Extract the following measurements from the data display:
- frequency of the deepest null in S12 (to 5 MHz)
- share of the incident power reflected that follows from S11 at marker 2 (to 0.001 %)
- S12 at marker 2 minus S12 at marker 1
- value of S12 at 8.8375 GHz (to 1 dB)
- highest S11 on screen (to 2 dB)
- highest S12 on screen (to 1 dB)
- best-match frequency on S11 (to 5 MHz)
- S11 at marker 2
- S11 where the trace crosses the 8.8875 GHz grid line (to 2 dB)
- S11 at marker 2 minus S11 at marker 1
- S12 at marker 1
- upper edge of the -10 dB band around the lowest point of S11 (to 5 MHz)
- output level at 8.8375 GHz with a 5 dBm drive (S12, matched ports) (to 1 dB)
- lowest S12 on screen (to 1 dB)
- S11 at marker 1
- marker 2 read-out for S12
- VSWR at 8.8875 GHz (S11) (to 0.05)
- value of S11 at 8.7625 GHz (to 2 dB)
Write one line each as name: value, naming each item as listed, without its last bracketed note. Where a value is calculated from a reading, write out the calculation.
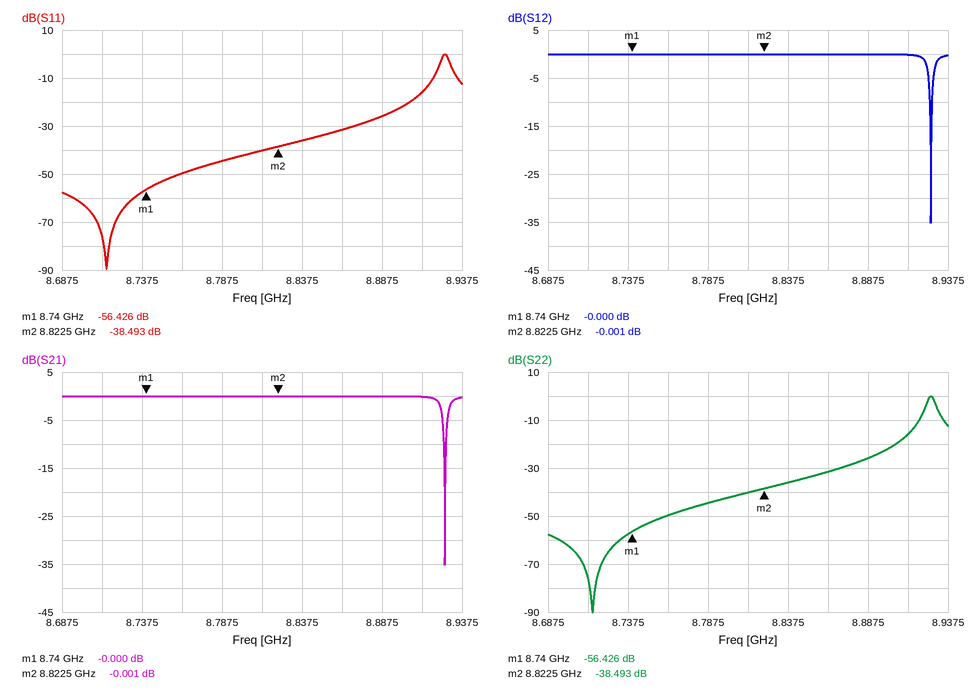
frequency of the deepest null in S12: 8.925 GHz
share of the incident power reflected that follows from S11 at marker 2: 10^(-38.493/10) ≈ 0.014 %
S12 at marker 2 minus S12 at marker 1: -0.001 − (-0) = -0.001 dB
value of S12 at 8.8375 GHz: 0 dB
highest S11 on screen: 0 dB
highest S12 on screen: 0 dB
best-match frequency on S11: 8.715 GHz
S11 at marker 2: -38.493 dB
S11 where the trace crosses the 8.8875 GHz grid line: -26 dB
S11 at marker 2 minus S11 at marker 1: -38.493 − (-56.426) = 17.933 dB
S12 at marker 1: -0.000 dB
upper edge of the -10 dB band around the lowest point of S11: 8.920 GHz
output level at 8.8375 GHz with a 5 dBm drive (S12, matched ports): 5 dBm + (0 dB) = 5 dBm
lowest S12 on screen: -35 dB
S11 at marker 1: -56.426 dB
marker 2 read-out for S12: -0.001 dB
VSWR at 8.8875 GHz (S11): |Γ| = 10^(-26/20) = 0.0501; VSWR = (1 + 0.0501)/(1 − 0.0501) ≈ 1.11, so 1.10 to the nearest 0.05
value of S11 at 8.7625 GHz: -50 dB
